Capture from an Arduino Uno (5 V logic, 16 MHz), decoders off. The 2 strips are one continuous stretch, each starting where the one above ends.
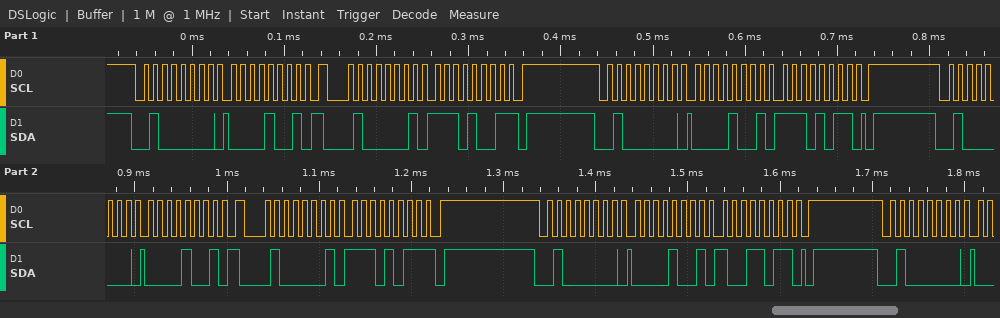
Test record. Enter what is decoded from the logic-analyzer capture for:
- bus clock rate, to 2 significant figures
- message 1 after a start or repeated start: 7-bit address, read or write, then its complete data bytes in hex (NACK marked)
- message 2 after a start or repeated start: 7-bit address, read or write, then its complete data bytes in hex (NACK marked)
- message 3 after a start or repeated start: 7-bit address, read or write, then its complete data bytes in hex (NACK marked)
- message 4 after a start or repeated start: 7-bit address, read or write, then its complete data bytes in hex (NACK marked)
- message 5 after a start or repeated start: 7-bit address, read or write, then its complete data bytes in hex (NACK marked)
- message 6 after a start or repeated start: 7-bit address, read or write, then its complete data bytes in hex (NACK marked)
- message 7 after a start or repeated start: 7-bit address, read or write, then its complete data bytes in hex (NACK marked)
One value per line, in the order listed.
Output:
100 kHz
0x20 write: 09
0x20 read: E9 NACK
0x20 write: 09 EB
0x20 write: 09
0x20 read: EB NACK
0x20 write: 09 9B
0x20 write
